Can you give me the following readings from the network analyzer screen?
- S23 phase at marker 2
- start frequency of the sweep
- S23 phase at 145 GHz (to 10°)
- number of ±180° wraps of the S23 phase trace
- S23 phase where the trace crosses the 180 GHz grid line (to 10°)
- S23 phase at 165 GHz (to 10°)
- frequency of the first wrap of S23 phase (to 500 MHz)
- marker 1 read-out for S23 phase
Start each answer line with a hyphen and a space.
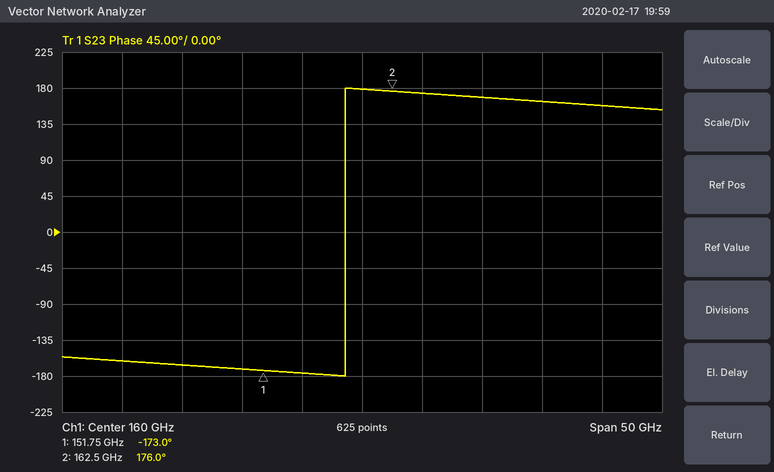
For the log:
- 176.0°
- 135 GHz
- -170°
- 1
- 160°
- 170°
- 158.5 GHz
- -173.0°
